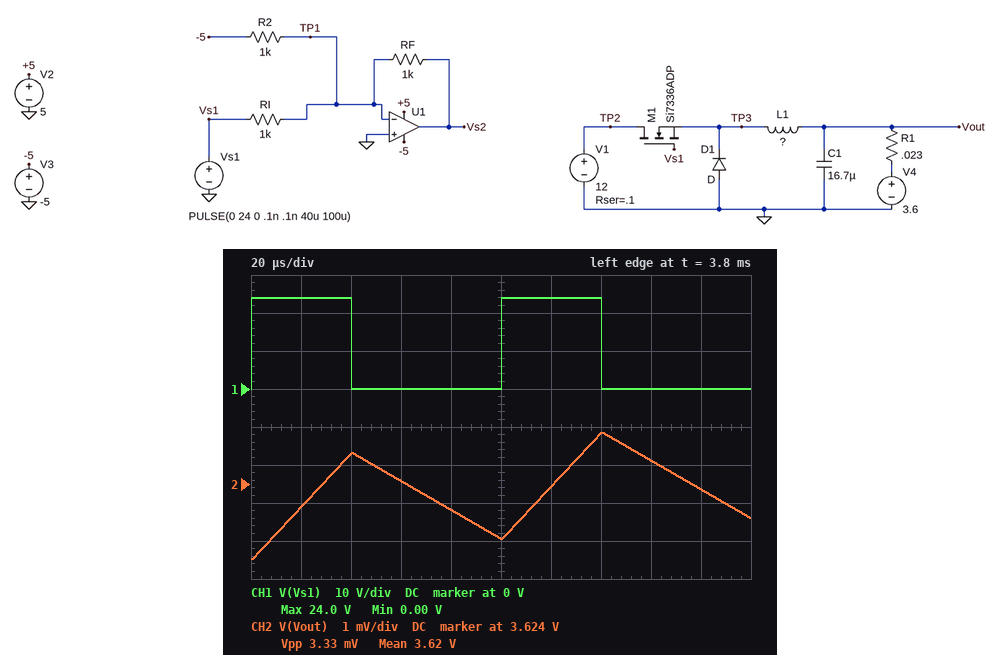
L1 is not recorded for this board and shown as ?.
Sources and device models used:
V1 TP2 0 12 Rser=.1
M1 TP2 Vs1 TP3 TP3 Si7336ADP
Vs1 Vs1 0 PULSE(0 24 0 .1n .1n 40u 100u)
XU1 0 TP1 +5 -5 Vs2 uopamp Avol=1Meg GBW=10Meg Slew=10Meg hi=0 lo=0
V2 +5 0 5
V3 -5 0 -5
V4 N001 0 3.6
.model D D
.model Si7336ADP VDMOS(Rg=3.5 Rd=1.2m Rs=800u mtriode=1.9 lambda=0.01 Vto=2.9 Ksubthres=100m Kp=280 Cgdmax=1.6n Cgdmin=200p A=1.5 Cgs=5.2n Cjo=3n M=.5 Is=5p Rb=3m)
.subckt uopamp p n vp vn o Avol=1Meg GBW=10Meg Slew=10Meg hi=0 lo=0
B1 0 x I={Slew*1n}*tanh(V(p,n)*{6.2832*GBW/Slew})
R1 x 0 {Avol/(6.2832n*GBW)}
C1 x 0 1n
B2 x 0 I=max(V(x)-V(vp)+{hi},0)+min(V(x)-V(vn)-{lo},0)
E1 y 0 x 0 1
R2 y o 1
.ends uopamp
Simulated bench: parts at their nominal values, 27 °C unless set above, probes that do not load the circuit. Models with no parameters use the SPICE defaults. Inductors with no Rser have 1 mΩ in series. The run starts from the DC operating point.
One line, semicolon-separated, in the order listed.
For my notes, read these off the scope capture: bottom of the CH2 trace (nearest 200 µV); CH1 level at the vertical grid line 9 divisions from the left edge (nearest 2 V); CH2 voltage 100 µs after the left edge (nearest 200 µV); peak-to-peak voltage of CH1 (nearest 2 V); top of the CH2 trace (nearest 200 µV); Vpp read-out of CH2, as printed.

3.6220 V; 0 V; 3.6226 V; 24 V; 3.6254 V; 3.33 mV
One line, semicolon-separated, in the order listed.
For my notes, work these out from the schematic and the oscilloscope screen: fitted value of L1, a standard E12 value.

2.7 mH
